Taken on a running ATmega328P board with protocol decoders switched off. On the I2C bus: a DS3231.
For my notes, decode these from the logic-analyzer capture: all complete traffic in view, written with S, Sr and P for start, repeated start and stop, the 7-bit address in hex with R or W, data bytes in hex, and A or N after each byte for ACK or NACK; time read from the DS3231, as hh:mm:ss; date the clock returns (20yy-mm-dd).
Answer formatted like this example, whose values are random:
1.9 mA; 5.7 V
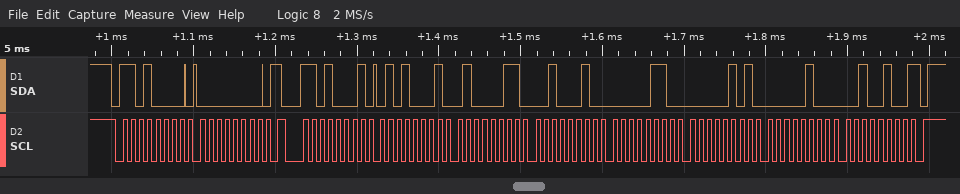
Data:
S 68W A 00 A Sr 68R A 51 A 43 A 22 A 06 A 05 A 04 A 24 N P; 22:43:51; 2024-04-05
